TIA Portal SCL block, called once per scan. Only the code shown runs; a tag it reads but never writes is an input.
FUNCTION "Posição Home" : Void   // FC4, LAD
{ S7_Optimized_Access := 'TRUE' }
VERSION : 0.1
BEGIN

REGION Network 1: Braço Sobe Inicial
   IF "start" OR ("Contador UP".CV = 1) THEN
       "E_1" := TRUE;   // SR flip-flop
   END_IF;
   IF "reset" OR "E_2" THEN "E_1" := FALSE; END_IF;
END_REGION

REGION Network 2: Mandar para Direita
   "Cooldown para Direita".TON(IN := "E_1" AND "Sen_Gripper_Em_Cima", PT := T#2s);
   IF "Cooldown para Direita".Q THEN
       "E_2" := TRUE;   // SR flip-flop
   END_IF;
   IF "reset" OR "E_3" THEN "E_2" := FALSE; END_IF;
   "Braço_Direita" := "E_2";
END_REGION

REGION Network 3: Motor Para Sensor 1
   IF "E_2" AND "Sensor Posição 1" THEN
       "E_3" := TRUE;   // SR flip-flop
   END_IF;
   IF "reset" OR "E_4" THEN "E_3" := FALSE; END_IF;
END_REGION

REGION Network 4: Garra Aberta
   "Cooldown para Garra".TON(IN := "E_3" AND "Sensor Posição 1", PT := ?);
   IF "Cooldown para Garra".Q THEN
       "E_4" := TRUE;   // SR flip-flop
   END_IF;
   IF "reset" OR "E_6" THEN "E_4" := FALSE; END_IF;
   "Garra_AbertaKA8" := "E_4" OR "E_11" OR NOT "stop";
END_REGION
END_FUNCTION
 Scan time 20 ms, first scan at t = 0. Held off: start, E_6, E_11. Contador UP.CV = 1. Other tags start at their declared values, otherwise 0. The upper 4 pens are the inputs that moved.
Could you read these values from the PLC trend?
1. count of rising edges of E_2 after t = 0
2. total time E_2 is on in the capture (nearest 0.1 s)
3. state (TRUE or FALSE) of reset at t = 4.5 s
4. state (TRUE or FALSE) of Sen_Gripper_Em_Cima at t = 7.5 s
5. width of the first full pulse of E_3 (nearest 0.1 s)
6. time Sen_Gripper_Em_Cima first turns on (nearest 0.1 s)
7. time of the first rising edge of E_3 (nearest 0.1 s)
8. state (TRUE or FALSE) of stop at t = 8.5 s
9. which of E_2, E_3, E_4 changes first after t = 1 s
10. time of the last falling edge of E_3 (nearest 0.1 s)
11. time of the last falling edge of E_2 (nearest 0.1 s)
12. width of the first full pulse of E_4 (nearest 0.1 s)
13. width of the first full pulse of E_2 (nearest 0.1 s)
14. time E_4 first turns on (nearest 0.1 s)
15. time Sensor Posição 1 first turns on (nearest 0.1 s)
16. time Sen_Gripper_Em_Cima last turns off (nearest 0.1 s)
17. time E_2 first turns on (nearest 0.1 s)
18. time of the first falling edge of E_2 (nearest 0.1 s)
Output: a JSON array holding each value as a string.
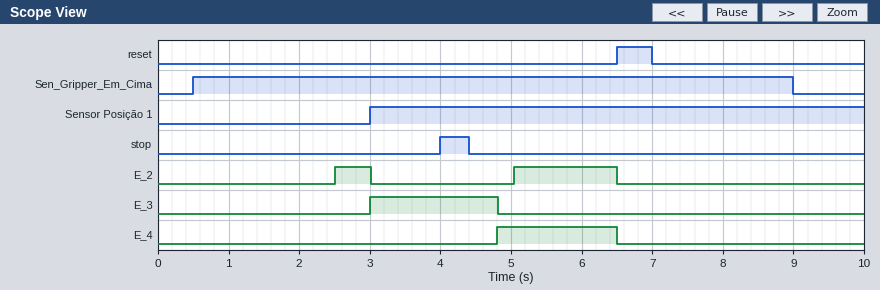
["2", "2.0 s", "FALSE", "TRUE", "1.8 s", "0.5 s", "3.0 s", "FALSE", "E_2", "4.8 s", "6.5 s", "1.7 s", "0.5 s", "4.8 s", "3.0 s", "9.0 s", "2.5 s", "3.0 s"]
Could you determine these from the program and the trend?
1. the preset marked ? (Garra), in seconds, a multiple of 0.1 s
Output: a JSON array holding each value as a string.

["1.8 s"]
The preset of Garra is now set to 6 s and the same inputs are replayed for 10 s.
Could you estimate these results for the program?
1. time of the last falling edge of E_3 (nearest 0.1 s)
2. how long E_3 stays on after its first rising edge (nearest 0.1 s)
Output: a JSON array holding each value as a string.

["6.5 s", "3.5 s"]
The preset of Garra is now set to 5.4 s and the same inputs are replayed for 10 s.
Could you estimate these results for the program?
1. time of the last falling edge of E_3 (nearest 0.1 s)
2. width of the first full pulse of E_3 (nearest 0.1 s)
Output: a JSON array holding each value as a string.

["6.5 s", "3.5 s"]
